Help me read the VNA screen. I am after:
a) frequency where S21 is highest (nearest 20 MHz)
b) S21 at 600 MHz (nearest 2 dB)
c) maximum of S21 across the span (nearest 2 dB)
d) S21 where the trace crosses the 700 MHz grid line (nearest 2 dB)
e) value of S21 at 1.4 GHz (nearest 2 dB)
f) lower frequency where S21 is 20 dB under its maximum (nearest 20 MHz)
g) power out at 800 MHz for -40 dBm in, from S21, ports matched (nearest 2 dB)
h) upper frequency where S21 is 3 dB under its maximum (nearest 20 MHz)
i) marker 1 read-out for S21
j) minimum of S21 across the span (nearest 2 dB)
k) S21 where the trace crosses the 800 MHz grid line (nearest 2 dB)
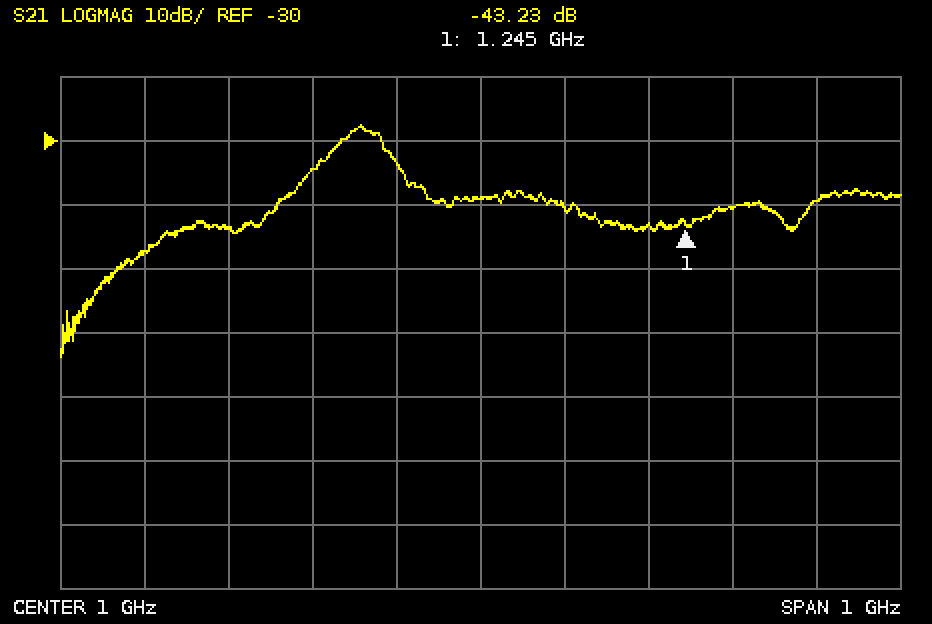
860 MHz
-48 dB
-28 dB
-44 dB
-40 dB
600 MHz
-74 dBm
880 MHz
-43.23 dB
-64 dB
-34 dB
